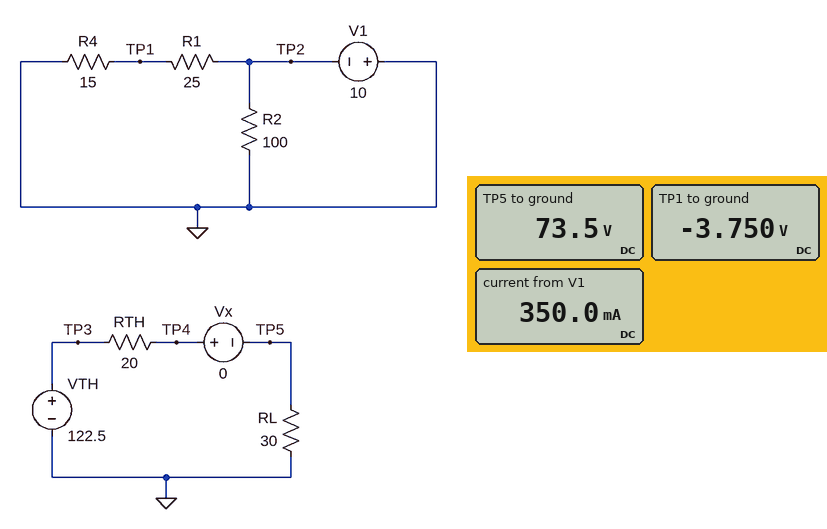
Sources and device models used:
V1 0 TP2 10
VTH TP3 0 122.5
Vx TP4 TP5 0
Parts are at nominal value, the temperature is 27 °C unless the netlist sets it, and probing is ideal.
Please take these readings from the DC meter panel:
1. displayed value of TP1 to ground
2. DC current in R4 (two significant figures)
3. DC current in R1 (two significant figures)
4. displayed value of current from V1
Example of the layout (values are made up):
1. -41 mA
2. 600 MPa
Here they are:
1. -3.750 V
2. 250 mA
3. 250 mA
4. 350.0 mA
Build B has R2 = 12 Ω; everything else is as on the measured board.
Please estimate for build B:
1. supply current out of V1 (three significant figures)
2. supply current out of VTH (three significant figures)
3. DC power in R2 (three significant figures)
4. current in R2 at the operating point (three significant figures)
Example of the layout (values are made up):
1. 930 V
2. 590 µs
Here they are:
1. 1.08 A
2. 2.45 A
3. 8.33 W
4. 833 mA
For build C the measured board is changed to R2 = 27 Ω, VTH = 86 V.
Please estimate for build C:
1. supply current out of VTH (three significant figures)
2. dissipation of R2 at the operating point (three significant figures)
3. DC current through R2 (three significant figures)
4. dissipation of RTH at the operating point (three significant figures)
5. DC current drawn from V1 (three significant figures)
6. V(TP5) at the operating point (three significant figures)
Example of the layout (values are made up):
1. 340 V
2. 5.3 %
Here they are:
1. 1.72 A
2. 3.70 W
3. 370 mA
4. 59.2 W
5. 620 mA
6. 51.6 V
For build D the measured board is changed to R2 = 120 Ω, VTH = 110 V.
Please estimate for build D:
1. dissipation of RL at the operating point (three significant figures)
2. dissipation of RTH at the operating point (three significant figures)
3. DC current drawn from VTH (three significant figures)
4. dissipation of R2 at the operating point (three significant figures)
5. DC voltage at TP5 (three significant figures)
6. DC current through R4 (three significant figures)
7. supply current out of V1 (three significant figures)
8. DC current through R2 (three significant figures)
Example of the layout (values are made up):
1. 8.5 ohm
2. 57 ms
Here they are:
1. 145 W
2. 96.8 W
3. 2.20 A
4. 833 mW
5. 66.0 V
6. 250 mA
7. 333 mA
8. 83.3 mA
